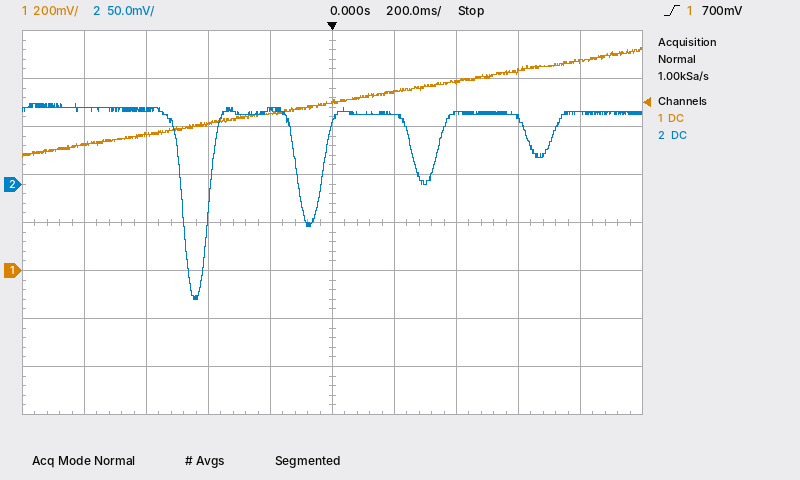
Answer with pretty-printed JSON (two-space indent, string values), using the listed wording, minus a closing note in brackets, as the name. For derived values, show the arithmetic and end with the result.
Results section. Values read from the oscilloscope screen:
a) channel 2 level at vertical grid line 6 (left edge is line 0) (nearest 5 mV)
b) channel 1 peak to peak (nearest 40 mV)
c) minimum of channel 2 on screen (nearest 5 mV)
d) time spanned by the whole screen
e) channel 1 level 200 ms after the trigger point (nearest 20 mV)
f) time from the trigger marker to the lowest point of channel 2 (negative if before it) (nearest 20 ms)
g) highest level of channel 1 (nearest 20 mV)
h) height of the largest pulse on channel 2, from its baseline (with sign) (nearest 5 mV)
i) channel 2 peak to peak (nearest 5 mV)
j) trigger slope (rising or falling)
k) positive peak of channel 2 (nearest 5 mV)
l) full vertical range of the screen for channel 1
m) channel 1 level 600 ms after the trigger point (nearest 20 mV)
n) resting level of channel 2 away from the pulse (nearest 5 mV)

{
  "channel 2 level at vertical grid line 6 (left edge is line 0)": "70 mV",
  "channel 1 peak to peak": "440 mV",
  "minimum of channel 2 on screen": "-120 mV",
  "time spanned by the whole screen": "2 s",
  "channel 1 level 200 ms after the trigger point": "740 mV",
  "time from the trigger marker to the lowest point of channel 2 (negative if before it)": "-440 ms",
  "highest level of channel 1": "920 mV",
  "height of the largest pulse on channel 2, from its baseline (with sign)": "-120 mV − (75 mV) = -195 mV",
  "channel 2 peak to peak": "85 mV − (-120 mV) = 205 mV",
  "trigger slope": "rising",
  "positive peak of channel 2": "85 mV",
  "full vertical range of the screen for channel 1": "1.6 V",
  "channel 1 level 600 ms after the trigger point": "820 mV",
  "resting level of channel 2 away from the pulse": "75 mV"
}
